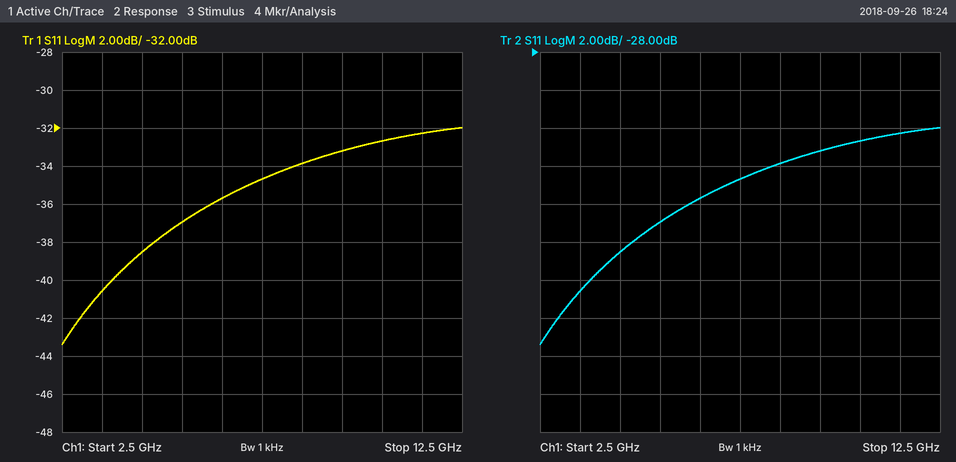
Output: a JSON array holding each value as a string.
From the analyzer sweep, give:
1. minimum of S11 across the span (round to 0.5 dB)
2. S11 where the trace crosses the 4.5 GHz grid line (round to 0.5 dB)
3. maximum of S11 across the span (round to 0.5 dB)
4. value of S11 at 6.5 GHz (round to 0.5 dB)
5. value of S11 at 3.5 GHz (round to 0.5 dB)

["-43.5 dB", "-38.5 dB", "-32.0 dB", "-35.5 dB", "-40.5 dB"]
